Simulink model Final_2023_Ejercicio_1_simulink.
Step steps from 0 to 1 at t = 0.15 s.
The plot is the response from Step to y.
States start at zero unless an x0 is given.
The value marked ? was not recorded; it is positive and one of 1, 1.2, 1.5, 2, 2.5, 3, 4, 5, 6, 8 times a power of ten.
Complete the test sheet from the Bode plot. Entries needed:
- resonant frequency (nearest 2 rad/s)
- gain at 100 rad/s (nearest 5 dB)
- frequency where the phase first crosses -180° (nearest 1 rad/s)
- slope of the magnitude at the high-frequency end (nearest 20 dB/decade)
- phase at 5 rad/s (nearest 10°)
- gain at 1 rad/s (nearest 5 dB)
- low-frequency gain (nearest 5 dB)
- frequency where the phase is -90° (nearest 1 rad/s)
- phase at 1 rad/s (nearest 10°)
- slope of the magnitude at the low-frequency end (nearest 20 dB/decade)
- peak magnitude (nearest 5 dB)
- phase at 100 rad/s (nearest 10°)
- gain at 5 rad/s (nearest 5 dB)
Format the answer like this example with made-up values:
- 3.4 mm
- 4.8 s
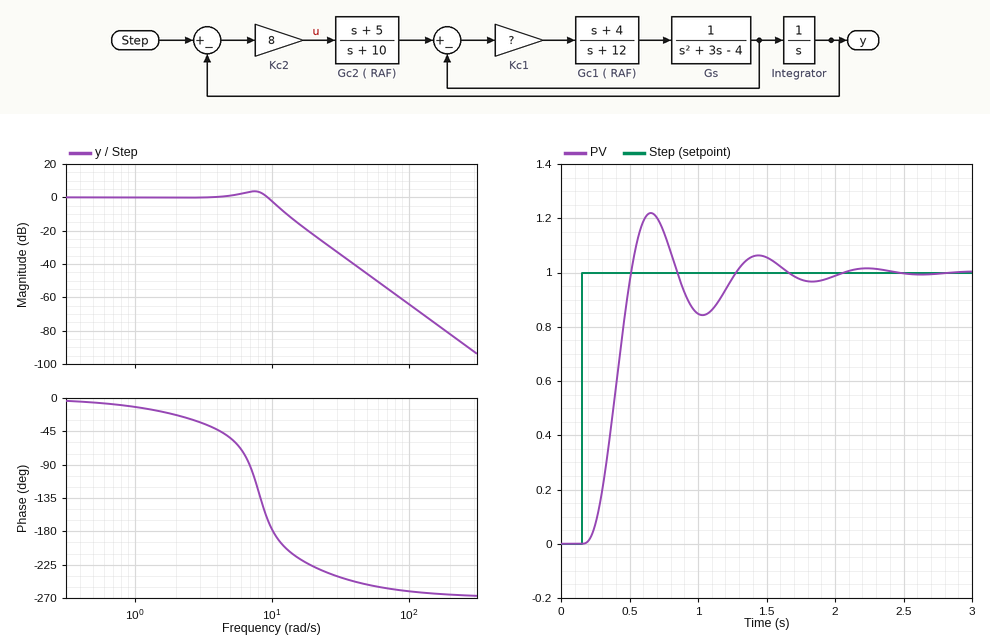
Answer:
- 8 rad/s
- -65 dB
- 10 rad/s
- -60 dB/decade
- -50°
- 0 dB
- 0 dB
- 7 rad/s
- -10°
- 0 dB/decade
- 5 dB
- -260°
- 0 dB
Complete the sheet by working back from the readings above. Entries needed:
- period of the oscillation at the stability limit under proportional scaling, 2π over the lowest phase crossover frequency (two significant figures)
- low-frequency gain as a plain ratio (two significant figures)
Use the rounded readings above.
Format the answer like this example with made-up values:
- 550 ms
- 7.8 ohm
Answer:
- 0.63 s
- 1.0
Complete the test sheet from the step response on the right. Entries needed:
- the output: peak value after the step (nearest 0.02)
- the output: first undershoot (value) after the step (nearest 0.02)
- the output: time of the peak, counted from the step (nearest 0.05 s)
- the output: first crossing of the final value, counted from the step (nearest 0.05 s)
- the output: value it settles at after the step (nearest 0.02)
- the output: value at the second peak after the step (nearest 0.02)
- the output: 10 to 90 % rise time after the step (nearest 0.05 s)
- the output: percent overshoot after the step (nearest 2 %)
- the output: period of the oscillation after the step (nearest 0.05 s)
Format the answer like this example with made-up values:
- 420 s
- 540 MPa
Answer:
- 1.22
- 0.84
- 0.50 s
- 0.35 s
- 1.00
- 1.06
- 0.20 s
- 22 %
- 0.80 s
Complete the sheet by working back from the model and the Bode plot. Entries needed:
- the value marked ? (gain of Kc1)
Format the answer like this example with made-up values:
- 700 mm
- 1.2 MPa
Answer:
- 80
